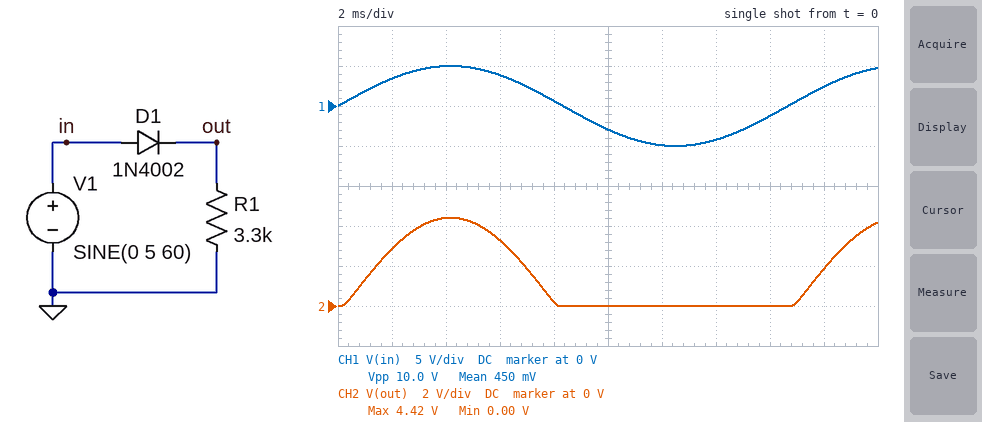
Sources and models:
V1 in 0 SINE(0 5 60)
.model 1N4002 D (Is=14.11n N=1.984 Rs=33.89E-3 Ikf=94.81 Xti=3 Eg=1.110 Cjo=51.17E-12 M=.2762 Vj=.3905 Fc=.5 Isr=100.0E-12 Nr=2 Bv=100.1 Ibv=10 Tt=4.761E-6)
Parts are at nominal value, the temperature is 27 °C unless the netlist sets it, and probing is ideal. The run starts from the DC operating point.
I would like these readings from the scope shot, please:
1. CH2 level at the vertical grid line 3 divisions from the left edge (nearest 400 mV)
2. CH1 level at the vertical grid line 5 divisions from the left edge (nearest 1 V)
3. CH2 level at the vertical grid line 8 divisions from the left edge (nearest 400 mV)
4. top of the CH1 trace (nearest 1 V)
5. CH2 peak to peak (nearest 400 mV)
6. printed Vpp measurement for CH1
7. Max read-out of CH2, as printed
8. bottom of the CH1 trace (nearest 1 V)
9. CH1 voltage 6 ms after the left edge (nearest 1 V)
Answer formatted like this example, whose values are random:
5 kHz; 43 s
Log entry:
3.2 V; -3 V; 0 V; 5 V; 4.4 V; 10.0 V; 4.42 V; -5 V; 4 V
